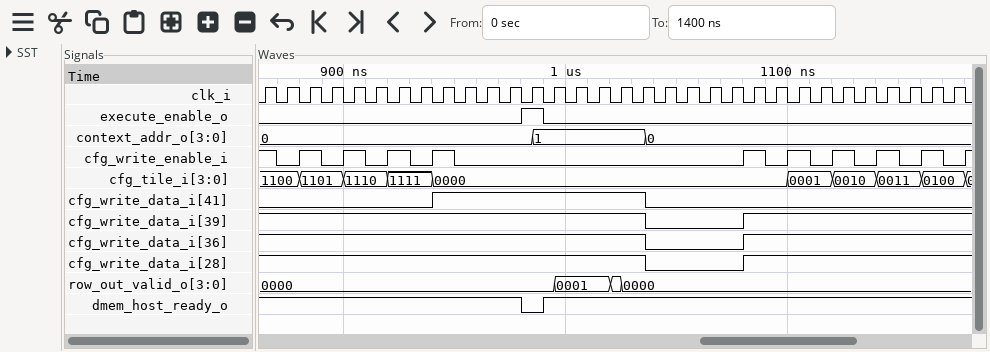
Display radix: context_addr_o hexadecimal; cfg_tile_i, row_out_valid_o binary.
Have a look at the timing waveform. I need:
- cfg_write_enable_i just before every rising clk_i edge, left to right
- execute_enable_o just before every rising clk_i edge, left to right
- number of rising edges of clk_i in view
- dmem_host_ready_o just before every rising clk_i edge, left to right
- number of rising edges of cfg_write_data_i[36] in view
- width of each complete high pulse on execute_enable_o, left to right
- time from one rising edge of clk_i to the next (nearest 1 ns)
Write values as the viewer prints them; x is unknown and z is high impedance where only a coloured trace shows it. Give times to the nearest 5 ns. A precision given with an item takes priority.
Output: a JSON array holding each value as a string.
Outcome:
["1 0 1 0 1 0 1 0 1 0 0 0 0 0 0 0 0 0 0 0 0 0 1 0 1 0 1 0 1 0 1 0", "0 0 0 0 0 0 0 0 0 0 0 0 1 0 0 0 0 0 0 0 0 0 0 0 0 0 0 0 0 0 0 0", "32", "1 1 1 1 1 1 1 1 1 1 1 1 0 1 1 1 1 1 1 1 1 1 1 1 1 1 1 1 1 1 1 1", "1", "10 ns", "10 ns"]
